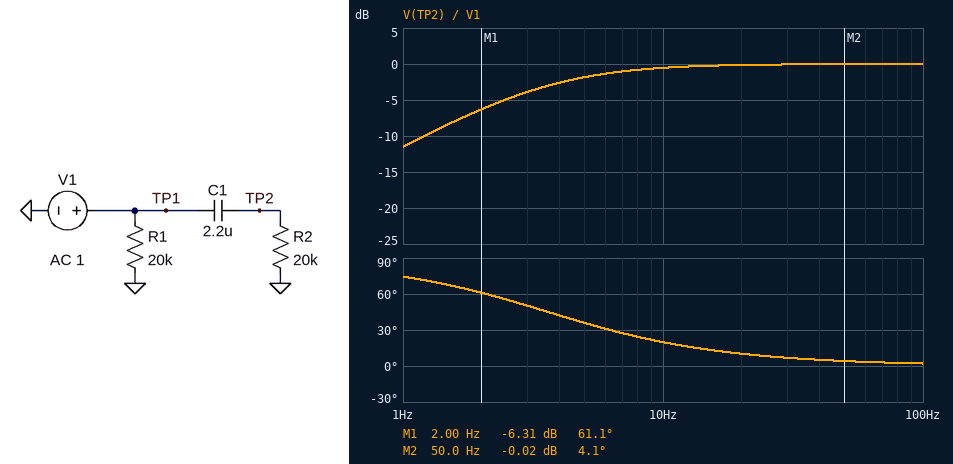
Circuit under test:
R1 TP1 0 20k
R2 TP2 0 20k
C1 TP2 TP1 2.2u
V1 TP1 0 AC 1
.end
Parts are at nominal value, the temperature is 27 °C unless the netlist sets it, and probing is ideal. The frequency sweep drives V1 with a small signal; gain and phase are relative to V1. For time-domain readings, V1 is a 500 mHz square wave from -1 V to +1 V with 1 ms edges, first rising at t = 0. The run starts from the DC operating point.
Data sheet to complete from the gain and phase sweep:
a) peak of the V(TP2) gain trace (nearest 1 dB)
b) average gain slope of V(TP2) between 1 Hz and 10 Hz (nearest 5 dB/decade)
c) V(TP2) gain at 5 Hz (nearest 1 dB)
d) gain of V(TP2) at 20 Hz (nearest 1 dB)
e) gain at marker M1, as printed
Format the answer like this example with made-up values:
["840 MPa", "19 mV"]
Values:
["0 dB", "10 dB/decade", "-2 dB", "0 dB", "-6.31 dB"]
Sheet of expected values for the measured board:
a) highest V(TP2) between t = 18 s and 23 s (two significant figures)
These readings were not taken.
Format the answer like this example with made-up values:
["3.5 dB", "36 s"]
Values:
["2.0 V"]
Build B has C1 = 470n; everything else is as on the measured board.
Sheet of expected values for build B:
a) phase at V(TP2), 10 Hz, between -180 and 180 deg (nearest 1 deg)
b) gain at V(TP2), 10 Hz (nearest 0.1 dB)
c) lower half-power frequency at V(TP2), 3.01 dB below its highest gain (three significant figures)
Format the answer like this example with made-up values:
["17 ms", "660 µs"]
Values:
["59 deg", "-5.9 dB", "16.9 Hz"]
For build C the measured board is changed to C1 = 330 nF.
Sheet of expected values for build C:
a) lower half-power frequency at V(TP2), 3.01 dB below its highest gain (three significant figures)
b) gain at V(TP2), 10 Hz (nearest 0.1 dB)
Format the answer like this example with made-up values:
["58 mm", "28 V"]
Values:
["24.1 Hz", "-8.3 dB"]
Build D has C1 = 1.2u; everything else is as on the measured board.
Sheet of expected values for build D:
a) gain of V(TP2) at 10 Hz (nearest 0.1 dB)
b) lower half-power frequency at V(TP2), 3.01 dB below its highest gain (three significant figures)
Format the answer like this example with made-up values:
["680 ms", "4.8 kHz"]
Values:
["-1.6 dB", "6.63 Hz"]
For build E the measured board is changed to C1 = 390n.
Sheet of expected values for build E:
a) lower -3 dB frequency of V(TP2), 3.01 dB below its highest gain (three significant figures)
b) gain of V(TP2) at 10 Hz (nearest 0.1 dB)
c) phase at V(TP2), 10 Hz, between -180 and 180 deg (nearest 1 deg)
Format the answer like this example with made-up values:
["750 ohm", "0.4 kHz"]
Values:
["20.4 Hz", "-7.1 dB", "64 deg"]
